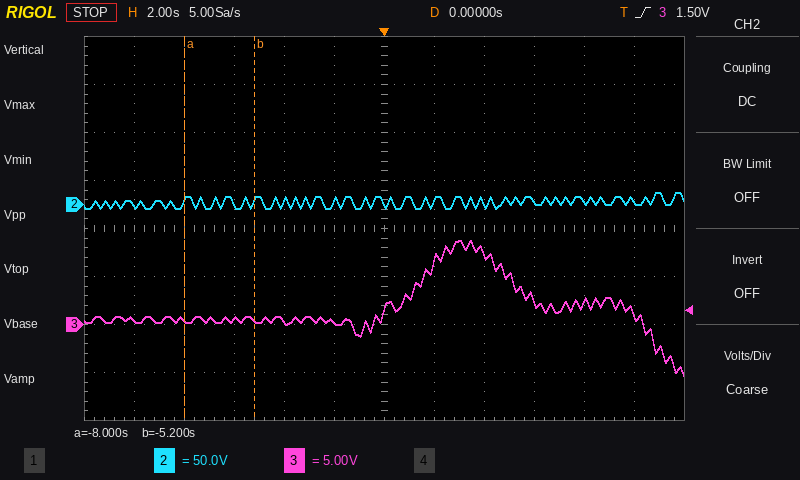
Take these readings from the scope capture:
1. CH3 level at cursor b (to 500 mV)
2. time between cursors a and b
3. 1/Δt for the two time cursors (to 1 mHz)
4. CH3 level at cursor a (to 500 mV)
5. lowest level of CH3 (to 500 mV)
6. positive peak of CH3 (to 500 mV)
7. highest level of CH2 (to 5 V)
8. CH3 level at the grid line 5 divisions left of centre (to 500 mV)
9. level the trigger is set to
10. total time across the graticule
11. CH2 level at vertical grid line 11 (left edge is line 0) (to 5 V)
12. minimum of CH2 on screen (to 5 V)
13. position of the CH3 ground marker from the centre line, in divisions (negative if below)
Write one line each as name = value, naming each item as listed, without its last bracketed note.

CH3 level at cursor b = 500 mV
time between cursors a and b = 2.8 s
1/Δt for the two time cursors = 357 mHz
CH3 level at cursor a = 500 mV
lowest level of CH3 = -5.5 V
positive peak of CH3 = 9.0 V
highest level of CH2 = 10 V
CH3 level at the grid line 5 divisions left of centre = 500 mV
level the trigger is set to = 1.50 V
total time across the graticule = 24 s
CH2 level at vertical grid line 11 (left edge is line 0) = 5 V
minimum of CH2 on screen = -5 V
position of the CH3 ground marker from the centre line, in divisions = -2.0 div
